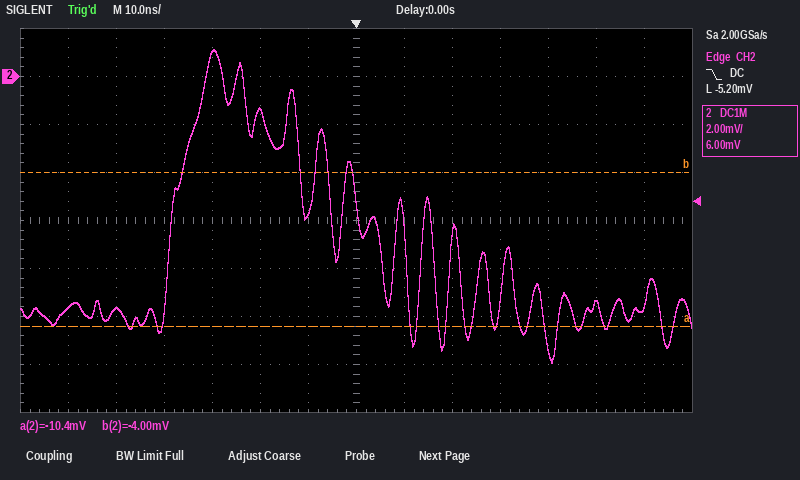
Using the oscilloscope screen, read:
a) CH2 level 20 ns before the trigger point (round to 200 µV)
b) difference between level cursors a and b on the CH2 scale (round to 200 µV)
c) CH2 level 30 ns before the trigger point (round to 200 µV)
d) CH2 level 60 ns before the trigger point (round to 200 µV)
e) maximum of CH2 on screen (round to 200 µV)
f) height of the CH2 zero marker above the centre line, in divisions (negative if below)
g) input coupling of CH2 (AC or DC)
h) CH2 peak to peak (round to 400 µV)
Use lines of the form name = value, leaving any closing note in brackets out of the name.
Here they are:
CH2 level 20 ns before the trigger point = -1.4 mV
difference between level cursors a and b on the CH2 scale = 6.4 mV
CH2 level 30 ns before the trigger point = 1.0 mV
CH2 level 60 ns before the trigger point = -9.6 mV
maximum of CH2 on screen = 1.2 mV
height of the CH2 zero marker above the centre line, in divisions = +3.0 div
input coupling of CH2 = DC
CH2 peak to peak = 13.2 mV
